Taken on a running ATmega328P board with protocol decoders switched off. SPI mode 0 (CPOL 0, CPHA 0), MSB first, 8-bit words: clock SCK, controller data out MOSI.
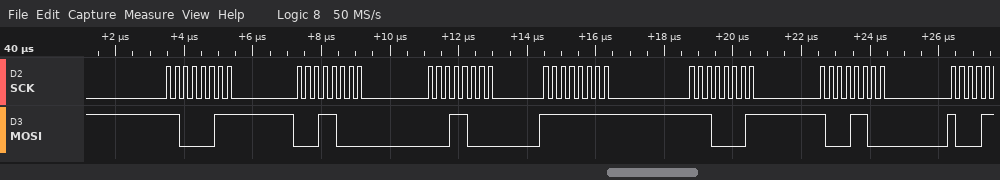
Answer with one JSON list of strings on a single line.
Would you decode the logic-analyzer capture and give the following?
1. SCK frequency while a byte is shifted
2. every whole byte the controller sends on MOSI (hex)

["4 MHz", "C3 18 18 FF E1 8C"]
